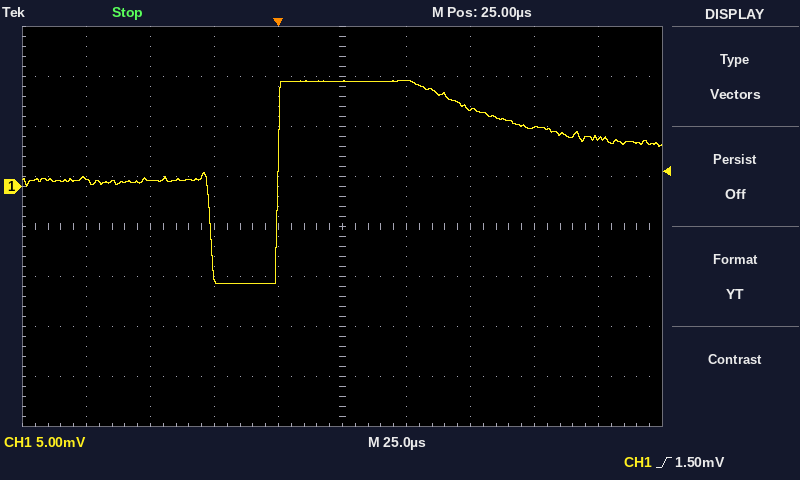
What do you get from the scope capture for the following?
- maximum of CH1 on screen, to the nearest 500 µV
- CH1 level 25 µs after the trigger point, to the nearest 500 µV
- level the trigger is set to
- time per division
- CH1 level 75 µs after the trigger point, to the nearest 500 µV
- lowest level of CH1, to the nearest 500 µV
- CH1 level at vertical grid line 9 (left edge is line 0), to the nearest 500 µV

10.5 mV
10.5 mV
1.50 mV
25 µs
7.5 mV
-9.5 mV
5.0 mV
